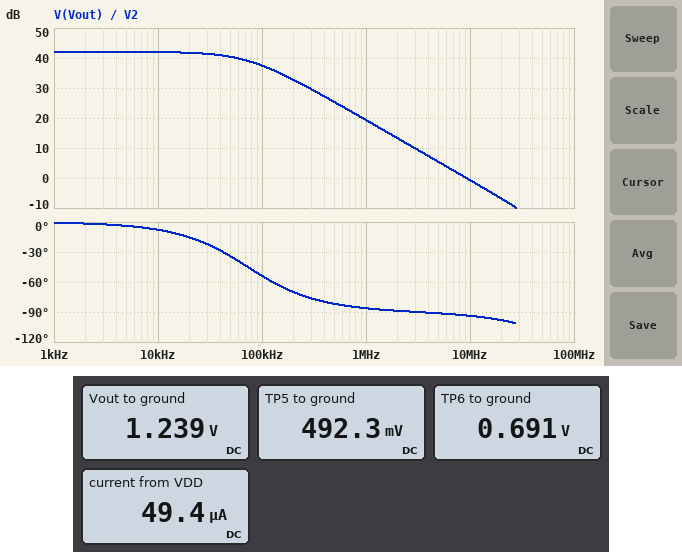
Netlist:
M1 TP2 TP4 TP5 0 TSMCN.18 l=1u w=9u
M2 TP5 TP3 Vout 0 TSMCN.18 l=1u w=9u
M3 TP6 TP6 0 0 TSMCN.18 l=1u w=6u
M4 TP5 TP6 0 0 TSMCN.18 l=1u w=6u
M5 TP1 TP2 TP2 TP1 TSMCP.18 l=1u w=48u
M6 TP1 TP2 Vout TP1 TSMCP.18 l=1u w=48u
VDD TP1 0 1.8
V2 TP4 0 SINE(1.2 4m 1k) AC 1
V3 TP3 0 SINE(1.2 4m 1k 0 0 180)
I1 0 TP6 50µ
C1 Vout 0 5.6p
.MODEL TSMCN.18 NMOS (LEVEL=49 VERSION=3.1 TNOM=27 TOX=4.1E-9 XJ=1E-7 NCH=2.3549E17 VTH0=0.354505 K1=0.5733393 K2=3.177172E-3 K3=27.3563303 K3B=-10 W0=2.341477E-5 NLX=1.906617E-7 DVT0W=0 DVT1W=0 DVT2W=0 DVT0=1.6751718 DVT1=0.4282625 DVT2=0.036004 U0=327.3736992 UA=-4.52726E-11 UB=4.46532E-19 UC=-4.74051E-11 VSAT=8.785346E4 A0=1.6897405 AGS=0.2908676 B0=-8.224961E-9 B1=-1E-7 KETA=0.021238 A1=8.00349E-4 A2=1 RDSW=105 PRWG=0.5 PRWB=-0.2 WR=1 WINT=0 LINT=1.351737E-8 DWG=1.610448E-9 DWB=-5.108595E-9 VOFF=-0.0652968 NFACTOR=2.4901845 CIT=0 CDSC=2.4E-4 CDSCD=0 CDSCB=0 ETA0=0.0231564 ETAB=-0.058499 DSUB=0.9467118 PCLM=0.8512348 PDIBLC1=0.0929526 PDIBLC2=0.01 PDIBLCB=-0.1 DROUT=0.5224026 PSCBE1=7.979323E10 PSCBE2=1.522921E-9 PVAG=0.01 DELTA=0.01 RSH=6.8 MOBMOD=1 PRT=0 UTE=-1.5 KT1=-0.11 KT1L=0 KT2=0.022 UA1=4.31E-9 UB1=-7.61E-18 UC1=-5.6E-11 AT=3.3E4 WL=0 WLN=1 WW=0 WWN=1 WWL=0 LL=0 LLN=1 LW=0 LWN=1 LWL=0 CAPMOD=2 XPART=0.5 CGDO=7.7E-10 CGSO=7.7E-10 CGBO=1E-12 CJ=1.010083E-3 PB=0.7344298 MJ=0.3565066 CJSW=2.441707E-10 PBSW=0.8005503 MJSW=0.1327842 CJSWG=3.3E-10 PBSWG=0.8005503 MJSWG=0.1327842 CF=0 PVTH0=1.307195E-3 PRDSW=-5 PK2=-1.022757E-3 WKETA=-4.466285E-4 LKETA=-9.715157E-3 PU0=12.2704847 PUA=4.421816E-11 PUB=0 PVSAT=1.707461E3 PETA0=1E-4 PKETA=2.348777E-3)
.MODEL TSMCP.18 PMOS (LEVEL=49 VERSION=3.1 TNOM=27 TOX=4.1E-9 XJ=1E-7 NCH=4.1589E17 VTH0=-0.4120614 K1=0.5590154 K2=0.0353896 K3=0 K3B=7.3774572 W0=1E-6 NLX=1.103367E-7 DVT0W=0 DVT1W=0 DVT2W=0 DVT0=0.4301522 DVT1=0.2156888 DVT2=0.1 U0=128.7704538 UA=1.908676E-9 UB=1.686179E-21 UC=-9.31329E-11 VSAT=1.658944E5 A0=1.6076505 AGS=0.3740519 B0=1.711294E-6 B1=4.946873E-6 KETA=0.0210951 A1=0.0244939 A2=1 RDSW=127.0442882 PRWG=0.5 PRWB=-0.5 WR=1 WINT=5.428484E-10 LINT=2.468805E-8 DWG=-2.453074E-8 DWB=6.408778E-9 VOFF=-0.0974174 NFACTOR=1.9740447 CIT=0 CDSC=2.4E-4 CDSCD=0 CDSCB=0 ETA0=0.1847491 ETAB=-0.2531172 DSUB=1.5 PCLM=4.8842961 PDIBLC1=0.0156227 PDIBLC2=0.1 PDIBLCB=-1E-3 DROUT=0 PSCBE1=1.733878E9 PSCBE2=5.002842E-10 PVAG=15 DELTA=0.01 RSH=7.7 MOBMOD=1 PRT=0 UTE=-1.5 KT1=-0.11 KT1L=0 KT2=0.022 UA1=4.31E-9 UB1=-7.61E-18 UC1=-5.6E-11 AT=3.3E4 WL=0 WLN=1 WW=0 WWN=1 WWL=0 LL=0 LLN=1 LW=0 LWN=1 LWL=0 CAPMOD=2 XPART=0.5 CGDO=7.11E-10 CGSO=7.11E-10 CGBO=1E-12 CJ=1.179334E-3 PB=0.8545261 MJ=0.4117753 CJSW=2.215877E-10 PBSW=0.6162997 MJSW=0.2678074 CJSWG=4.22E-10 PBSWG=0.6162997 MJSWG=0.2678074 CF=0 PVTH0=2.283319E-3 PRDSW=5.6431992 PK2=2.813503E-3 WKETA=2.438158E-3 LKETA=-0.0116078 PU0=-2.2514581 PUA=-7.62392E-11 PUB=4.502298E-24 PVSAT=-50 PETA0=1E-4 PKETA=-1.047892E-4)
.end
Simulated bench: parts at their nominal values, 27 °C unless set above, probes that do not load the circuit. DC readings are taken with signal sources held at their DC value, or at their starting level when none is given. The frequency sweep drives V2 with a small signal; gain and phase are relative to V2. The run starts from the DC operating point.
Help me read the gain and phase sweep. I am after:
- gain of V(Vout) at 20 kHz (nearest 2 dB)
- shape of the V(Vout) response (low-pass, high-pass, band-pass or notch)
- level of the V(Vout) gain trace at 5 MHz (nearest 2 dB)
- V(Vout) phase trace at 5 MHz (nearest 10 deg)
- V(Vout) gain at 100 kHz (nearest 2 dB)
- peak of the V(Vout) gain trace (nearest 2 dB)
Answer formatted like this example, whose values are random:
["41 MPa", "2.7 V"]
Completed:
["42 dB", "low-pass", "6 dB", "-90 deg", "38 dB", "42 dB"]
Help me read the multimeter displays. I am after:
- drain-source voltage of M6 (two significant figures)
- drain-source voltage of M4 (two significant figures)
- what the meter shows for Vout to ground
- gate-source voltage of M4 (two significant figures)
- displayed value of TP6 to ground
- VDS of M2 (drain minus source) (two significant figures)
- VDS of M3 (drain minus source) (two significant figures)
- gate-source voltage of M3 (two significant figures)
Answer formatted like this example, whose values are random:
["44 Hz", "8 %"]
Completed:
["560 mV", "490 mV", "1.239 V", "690 mV", "0.691 V", "-750 mV", "690 mV", "690 mV"]
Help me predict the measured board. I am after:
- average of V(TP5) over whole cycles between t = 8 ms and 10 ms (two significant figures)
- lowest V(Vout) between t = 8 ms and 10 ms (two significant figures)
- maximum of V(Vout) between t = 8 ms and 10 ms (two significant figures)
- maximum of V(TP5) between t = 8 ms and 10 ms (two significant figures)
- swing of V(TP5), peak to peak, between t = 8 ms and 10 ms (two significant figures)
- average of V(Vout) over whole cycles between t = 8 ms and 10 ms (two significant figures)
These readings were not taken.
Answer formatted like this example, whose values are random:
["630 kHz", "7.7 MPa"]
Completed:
["490 mV", "650 mV", "1.7 V", "490 mV", "3.5 mV", "1.2 V"]
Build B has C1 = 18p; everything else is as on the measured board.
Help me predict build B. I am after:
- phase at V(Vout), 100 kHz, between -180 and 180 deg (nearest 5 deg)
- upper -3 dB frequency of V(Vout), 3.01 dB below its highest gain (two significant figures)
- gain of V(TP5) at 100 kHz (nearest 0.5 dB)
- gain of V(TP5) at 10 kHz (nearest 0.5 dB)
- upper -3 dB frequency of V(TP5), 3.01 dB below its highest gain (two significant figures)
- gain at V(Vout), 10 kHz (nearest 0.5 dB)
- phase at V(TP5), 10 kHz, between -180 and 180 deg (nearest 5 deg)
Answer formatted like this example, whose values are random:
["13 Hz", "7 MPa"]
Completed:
["-75 deg", "23 kHz", "-7.5 dB", "-4.0 dB", "44 kHz", "41.5 dB", "-10 deg"]
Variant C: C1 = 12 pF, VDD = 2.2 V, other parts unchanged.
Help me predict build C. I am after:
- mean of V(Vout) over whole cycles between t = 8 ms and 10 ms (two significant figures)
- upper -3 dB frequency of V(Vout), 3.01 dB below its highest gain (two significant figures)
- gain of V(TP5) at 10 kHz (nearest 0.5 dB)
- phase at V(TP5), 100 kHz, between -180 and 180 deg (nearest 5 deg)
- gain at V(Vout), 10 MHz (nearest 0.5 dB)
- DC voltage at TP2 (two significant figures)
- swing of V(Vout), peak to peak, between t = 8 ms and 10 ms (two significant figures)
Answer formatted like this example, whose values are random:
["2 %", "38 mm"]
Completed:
["1.5 V", "33 kHz", "-4.0 dB", "-10 deg", "-7.0 dB", "1.6 V", "1.4 V"]
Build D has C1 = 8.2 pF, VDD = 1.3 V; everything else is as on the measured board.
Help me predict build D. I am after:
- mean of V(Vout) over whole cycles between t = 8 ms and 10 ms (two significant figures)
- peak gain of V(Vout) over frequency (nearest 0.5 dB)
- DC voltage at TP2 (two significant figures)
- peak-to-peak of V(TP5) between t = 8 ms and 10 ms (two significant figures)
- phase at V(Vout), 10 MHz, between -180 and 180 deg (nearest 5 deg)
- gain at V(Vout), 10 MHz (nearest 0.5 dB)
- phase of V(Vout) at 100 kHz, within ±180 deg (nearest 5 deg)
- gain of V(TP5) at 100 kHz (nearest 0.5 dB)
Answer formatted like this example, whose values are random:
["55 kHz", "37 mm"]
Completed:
["860 mV", "35.5 dB", "740 mV", "4.2 mV", "-95 deg", "-4.0 dB", "-45 deg", "-4.5 dB"]
